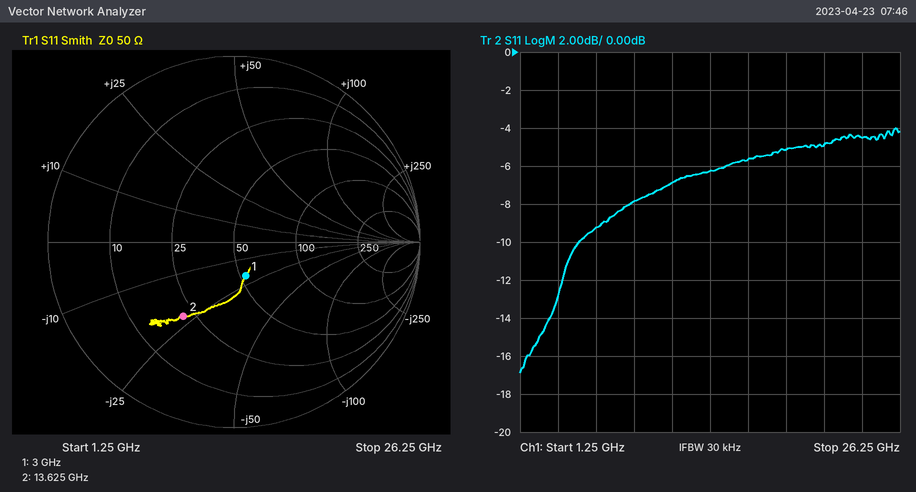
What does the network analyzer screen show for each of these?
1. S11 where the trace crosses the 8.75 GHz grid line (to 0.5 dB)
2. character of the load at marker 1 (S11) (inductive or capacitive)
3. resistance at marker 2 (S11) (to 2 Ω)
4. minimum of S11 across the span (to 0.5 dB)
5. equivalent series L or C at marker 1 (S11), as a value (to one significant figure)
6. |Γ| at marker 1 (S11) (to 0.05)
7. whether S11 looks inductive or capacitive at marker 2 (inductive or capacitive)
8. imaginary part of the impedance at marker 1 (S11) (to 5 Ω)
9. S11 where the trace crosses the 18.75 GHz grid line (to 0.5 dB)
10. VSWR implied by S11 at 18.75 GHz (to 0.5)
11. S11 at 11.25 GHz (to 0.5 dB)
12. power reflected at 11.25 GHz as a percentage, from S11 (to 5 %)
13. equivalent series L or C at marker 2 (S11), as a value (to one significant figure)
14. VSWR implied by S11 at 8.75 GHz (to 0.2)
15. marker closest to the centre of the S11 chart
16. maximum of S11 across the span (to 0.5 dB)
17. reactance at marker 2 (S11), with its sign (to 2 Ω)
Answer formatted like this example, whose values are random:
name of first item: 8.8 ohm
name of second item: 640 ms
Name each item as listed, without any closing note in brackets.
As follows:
S11 where the trace crosses the 8.75 GHz grid line: -8.0 dB
character of the load at marker 1 (S11): capacitive
resistance at marker 2 (S11): 22 Ω
minimum of S11 across the span: -17.0 dB
equivalent series L or C at marker 1 (S11), as a value: 3 pF
|Γ| at marker 1 (S11): 0.20
whether S11 looks inductive or capacitive at marker 2: capacitive
imaginary part of the impedance at marker 1 (S11): -20 Ω
S11 where the trace crosses the 18.75 GHz grid line: -5.0 dB
VSWR implied by S11 at 18.75 GHz: 3.5
S11 at 11.25 GHz: -7.0 dB
power reflected at 11.25 GHz as a percentage, from S11: 20 %
equivalent series L or C at marker 2 (S11), as a value: 500 fF
VSWR implied by S11 at 8.75 GHz: 2.4
marker closest to the centre of the S11 chart: marker 1
maximum of S11 across the span: -4.0 dB
reactance at marker 2 (S11), with its sign: -22 Ω
